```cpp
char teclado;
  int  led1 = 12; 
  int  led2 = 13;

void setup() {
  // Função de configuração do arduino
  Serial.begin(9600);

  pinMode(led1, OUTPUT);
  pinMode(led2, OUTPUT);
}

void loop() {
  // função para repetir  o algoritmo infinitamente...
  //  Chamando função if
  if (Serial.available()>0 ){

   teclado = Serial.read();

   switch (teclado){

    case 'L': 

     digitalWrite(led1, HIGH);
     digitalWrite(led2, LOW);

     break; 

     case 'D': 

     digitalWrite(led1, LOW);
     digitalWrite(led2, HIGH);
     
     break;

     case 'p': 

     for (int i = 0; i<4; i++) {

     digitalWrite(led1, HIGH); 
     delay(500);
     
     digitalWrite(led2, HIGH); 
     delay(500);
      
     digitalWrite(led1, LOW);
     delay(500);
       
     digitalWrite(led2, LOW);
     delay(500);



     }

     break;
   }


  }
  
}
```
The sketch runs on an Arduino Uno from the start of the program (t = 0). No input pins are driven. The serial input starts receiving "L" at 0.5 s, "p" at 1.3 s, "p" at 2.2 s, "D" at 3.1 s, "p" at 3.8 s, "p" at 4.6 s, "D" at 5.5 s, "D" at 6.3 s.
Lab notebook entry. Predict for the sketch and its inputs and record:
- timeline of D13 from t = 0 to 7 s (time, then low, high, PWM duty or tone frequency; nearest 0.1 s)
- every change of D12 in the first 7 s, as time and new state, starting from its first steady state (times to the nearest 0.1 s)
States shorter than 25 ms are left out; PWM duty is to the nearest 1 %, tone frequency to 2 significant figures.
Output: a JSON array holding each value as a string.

["0 s low; 1.8 s high; 2.8 s low; 3.8 s high; 4.8 s low; 5.8 s high; 6.8 s low", "0 s low; 0.5 s high; 2.3 s low; 3.3 s high; 4.3 s low; 5.3 s high; 6.3 s low"]
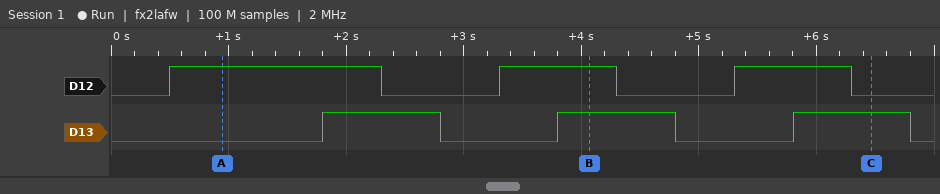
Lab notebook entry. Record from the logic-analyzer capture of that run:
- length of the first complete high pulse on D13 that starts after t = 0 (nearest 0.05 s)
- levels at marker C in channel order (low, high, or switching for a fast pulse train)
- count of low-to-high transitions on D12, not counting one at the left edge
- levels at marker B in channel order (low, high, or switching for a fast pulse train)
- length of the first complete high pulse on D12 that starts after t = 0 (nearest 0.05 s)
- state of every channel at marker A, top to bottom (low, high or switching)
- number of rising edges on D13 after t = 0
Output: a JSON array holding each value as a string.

["1.00 s", "D12 low, D13 high", "3", "D12 high, D13 high", "1.80 s", "D12 high, D13 low", "3"]
